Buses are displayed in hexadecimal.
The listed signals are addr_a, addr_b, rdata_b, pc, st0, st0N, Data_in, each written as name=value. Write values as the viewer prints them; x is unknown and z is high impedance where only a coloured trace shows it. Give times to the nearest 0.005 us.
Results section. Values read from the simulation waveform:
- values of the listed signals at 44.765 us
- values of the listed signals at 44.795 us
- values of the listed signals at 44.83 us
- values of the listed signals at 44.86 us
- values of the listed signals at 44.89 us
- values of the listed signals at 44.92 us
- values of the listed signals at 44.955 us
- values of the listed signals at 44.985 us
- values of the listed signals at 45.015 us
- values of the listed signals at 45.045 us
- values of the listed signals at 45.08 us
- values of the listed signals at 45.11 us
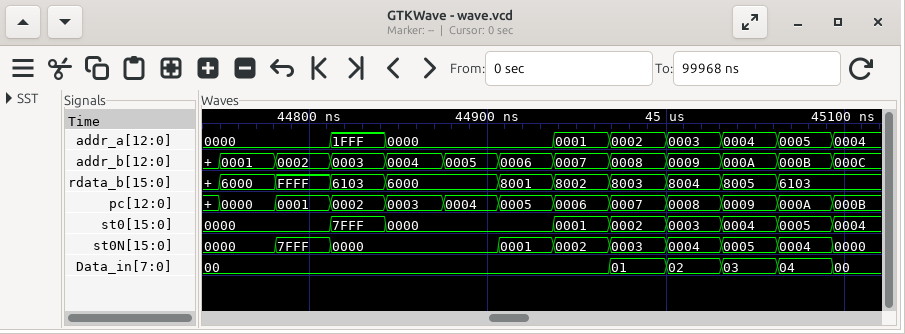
addr_a=0000, addr_b=0001, rdata_b=6000, pc=0000, st0=0000, st0N=0000, Data_in=00
addr_a=0000, addr_b=0002, rdata_b=FFFF, pc=0001, st0=0000, st0N=7FFF, Data_in=00
addr_a=1FFF, addr_b=0003, rdata_b=6103, pc=0002, st0=7FFF, st0N=0000, Data_in=00
addr_a=0000, addr_b=0004, rdata_b=6000, pc=0003, st0=0000, st0N=0000, Data_in=00
addr_a=0000, addr_b=0005, rdata_b=6000, pc=0004, st0=0000, st0N=0000, Data_in=00
addr_a=0000, addr_b=0006, rdata_b=8001, pc=0005, st0=0000, st0N=0001, Data_in=00
addr_a=0001, addr_b=0007, rdata_b=8002, pc=0006, st0=0001, st0N=0002, Data_in=00
addr_a=0002, addr_b=0008, rdata_b=8003, pc=0007, st0=0002, st0N=0003, Data_in=01
addr_a=0003, addr_b=0009, rdata_b=8004, pc=0008, st0=0003, st0N=0004, Data_in=02
addr_a=0004, addr_b=000A, rdata_b=8005, pc=0009, st0=0004, st0N=0005, Data_in=03
addr_a=0005, addr_b=000B, rdata_b=6103, pc=000A, st0=0005, st0N=0004, Data_in=04
addr_a=0004, addr_b=000C, rdata_b=6103, pc=000B, st0=0004, st0N=0000, Data_in=00
